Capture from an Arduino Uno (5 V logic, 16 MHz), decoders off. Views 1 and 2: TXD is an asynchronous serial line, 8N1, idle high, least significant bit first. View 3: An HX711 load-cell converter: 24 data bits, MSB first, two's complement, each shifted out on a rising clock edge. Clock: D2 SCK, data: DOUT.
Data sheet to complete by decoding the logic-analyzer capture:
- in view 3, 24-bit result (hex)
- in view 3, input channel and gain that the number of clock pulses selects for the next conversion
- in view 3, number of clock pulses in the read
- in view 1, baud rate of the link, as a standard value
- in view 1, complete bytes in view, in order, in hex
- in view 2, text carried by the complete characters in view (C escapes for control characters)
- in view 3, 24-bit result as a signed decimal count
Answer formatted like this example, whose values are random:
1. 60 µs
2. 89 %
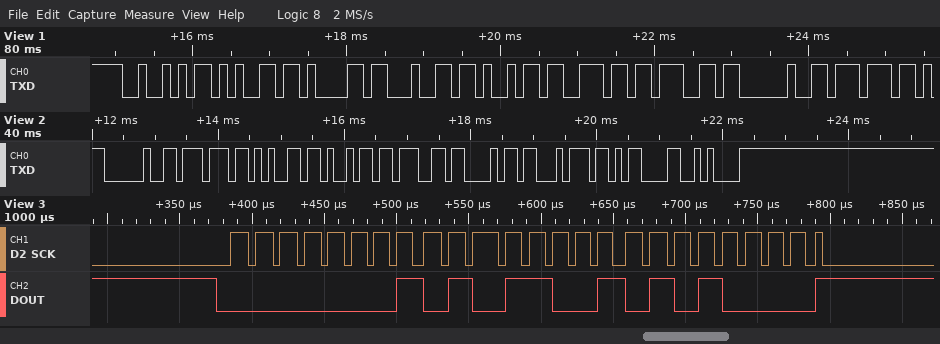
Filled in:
1. 0x015950
2. channel A, gain 128
3. 25
4. 9600 baud
5. 0x52 0x65 0x61 0x64 0x69 0x6E 0x67 0x20 0x77
6. " weight\r\n"
7. 88400
